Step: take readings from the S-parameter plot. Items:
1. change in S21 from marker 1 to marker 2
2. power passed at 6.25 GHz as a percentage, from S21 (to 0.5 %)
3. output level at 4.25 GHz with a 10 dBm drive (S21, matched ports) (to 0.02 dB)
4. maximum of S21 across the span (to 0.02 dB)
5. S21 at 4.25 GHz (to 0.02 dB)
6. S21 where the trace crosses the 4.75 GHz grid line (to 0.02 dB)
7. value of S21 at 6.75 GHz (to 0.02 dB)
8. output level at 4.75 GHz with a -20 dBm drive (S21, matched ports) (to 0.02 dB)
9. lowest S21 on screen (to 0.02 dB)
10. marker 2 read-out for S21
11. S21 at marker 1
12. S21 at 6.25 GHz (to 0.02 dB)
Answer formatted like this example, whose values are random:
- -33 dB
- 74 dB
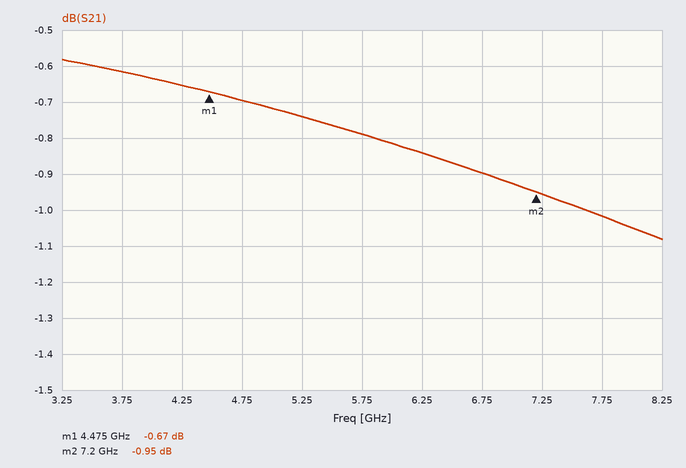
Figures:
- -0.28 dB
- 82.5 %
- 9.34 dBm
- -0.58 dB
- -0.66 dB
- -0.70 dB
- -0.90 dB
- -20.70 dBm
- -1.08 dB
- -0.95 dB
- -0.67 dB
- -0.84 dB
